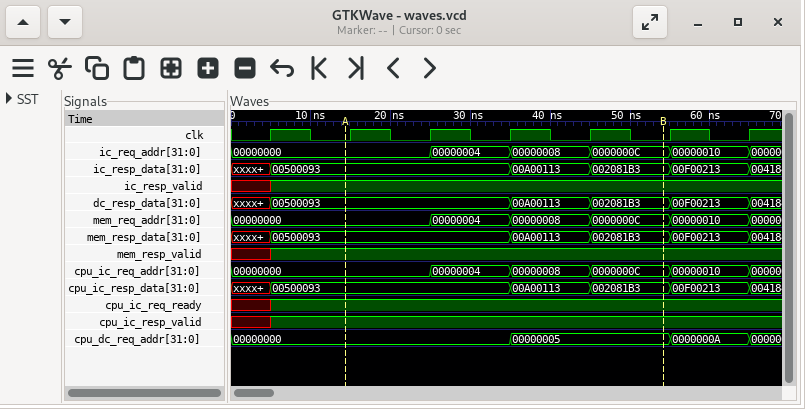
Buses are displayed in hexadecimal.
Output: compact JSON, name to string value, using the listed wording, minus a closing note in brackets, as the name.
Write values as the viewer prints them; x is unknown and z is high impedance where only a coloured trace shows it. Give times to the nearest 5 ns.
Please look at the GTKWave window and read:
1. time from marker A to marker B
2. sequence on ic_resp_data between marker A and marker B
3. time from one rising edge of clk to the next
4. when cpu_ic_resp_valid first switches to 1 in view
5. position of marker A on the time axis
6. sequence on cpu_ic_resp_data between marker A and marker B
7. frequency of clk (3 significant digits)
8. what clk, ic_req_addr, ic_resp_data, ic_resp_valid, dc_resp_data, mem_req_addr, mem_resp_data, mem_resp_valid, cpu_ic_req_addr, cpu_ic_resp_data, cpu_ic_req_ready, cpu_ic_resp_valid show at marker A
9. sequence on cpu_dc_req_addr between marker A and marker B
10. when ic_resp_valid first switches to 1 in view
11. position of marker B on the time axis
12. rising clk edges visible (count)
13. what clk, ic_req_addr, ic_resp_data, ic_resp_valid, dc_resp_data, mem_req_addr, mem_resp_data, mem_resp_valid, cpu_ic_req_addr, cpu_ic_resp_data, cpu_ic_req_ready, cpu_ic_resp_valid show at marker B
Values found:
{"time from marker A to marker B": "40 ns", "sequence on ic_resp_data between marker A and marker B": "00500093, 00A00113, 002081B3", "time from one rising edge of clk to the next": "10 ns", "when cpu_ic_resp_valid first switches to 1 in view": "5 ns", "position of marker A on the time axis": "15 ns", "sequence on cpu_ic_resp_data between marker A and marker B": "00500093, 00A00113, 002081B3", "frequency of clk": "100 MHz", "what clk, ic_req_addr, ic_resp_data, ic_resp_valid, dc_resp_data, mem_req_addr, mem_resp_data, mem_resp_valid, cpu_ic_req_addr, cpu_ic_resp_data, cpu_ic_req_ready, cpu_ic_resp_valid show at marker A": "clk=0, ic_req_addr=00000000, ic_resp_data=00500093, ic_resp_valid=1, dc_resp_data=00500093, mem_req_addr=00000000, mem_resp_data=00500093, mem_resp_valid=1, cpu_ic_req_addr=00000000, cpu_ic_resp_data=00500093, cpu_ic_req_ready=1, cpu_ic_resp_valid=1", "sequence on cpu_dc_req_addr between marker A and marker B": "00000000, 00000005", "when ic_resp_valid first switches to 1 in view": "5 ns", "position of marker B on the time axis": "55 ns", "rising clk edges visible": "7", "what clk, ic_req_addr, ic_resp_data, ic_resp_valid, dc_resp_data, mem_req_addr, mem_resp_data, mem_resp_valid, cpu_ic_req_addr, cpu_ic_resp_data, cpu_ic_req_ready, cpu_ic_resp_valid show at marker B": "clk=0, ic_req_addr=0000000C, ic_resp_data=002081B3, ic_resp_valid=1, dc_resp_data=002081B3, mem_req_addr=0000000C, mem_resp_data=002081B3, mem_resp_valid=1, cpu_ic_req_addr=0000000C, cpu_ic_resp_data=002081B3, cpu_ic_req_ready=1, cpu_ic_resp_valid=1"}
